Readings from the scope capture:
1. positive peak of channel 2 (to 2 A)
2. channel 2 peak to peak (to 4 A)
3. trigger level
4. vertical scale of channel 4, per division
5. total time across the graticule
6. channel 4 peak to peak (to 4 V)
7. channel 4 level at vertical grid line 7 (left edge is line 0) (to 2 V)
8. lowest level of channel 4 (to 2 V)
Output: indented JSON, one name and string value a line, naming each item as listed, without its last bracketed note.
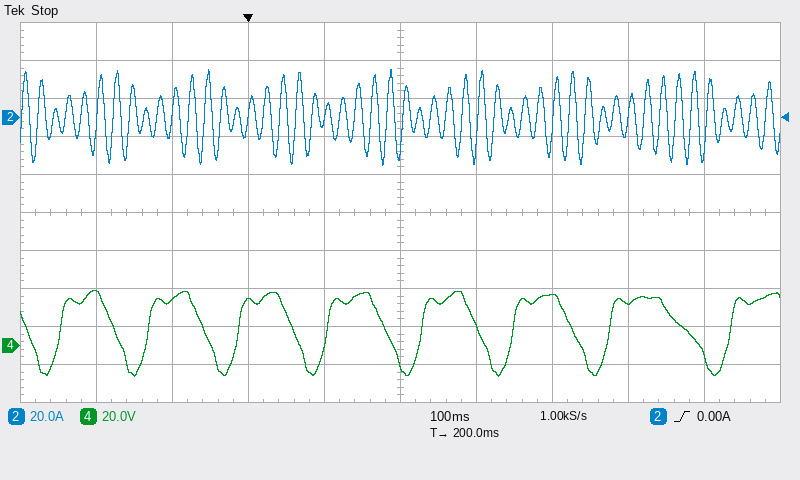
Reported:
{
  "positive peak of channel 2": "26 A",
  "channel 2 peak to peak": "52 A",
  "trigger level": "0.00 A",
  "vertical scale of channel 4, per division": "20 V",
  "total time across the graticule": "1 s",
  "channel 4 peak to peak": "44 V",
  "channel 4 level at vertical grid line 7 (left edge is line 0)": "26 V",
  "lowest level of channel 4": "-16 V"
}
